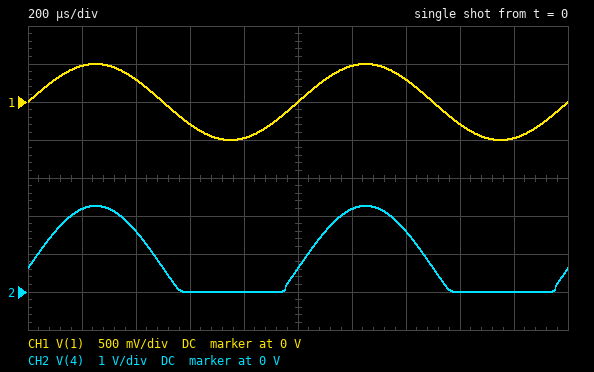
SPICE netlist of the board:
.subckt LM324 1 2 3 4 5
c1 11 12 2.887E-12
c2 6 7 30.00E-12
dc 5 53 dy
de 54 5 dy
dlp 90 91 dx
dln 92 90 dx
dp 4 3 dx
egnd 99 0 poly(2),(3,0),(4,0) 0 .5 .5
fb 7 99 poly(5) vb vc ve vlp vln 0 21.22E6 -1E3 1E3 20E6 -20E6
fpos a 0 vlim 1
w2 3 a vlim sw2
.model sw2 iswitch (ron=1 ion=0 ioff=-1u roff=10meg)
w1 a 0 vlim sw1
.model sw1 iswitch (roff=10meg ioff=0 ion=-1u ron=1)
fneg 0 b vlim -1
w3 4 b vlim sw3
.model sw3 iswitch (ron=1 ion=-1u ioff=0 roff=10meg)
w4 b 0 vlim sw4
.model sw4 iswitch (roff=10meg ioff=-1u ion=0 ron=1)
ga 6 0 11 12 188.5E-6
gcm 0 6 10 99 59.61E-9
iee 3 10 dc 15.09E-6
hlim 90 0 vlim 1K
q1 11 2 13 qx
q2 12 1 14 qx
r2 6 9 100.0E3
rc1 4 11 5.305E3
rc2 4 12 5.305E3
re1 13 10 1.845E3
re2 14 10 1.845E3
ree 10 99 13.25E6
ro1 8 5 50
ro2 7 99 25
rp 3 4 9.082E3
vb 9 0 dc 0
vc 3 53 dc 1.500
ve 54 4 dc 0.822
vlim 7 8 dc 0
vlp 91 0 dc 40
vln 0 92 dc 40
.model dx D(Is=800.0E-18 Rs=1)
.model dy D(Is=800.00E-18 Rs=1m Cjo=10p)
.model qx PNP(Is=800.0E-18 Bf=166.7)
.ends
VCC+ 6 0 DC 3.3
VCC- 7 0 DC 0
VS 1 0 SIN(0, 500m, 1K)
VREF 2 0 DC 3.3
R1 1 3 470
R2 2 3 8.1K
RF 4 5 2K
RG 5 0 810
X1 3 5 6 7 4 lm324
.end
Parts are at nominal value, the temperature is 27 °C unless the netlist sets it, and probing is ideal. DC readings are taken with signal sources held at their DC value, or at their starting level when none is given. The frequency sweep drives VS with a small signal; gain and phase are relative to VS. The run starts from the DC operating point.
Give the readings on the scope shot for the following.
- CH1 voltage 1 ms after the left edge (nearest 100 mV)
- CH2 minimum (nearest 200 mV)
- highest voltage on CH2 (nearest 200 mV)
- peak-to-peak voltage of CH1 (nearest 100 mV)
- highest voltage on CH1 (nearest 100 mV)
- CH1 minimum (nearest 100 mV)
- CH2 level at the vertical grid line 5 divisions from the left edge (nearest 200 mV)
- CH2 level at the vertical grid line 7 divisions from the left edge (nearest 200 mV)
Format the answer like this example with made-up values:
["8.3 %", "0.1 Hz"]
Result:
["0 V", "0 V", "2.2 V", "1.0 V", "500 mV", "-500 mV", "600 mV", "1.6 V"]
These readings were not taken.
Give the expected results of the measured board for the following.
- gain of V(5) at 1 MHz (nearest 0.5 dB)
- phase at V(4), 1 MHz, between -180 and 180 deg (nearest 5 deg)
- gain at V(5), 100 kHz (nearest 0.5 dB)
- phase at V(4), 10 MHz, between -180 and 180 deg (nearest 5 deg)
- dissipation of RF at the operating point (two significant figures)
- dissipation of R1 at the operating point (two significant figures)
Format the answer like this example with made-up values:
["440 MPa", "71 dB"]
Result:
["-11.5 dB", "-85 deg", "-1.0 dB", "-155 deg", "100 µW", "70 µW"]
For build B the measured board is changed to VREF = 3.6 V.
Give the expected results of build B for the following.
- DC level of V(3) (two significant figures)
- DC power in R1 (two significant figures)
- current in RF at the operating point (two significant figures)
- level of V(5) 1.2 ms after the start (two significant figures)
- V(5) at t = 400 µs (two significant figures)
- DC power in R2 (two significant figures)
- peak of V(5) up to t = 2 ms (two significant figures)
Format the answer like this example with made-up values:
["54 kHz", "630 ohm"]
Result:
["200 mV", "83 µW", "240 µA", "650 mV", "480 mV", "1.4 mW", "670 mV"]
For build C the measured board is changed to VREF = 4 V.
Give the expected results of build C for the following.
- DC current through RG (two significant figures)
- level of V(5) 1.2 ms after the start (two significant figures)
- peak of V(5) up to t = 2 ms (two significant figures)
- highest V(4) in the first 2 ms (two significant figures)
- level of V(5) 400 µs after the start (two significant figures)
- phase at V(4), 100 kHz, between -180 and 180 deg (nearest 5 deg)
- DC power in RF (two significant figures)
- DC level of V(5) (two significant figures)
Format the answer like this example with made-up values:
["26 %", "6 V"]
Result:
["270 µA", "670 mV", "690 mV", "2.4 V", "500 mV", "-20 deg", "150 µW", "220 mV"]
